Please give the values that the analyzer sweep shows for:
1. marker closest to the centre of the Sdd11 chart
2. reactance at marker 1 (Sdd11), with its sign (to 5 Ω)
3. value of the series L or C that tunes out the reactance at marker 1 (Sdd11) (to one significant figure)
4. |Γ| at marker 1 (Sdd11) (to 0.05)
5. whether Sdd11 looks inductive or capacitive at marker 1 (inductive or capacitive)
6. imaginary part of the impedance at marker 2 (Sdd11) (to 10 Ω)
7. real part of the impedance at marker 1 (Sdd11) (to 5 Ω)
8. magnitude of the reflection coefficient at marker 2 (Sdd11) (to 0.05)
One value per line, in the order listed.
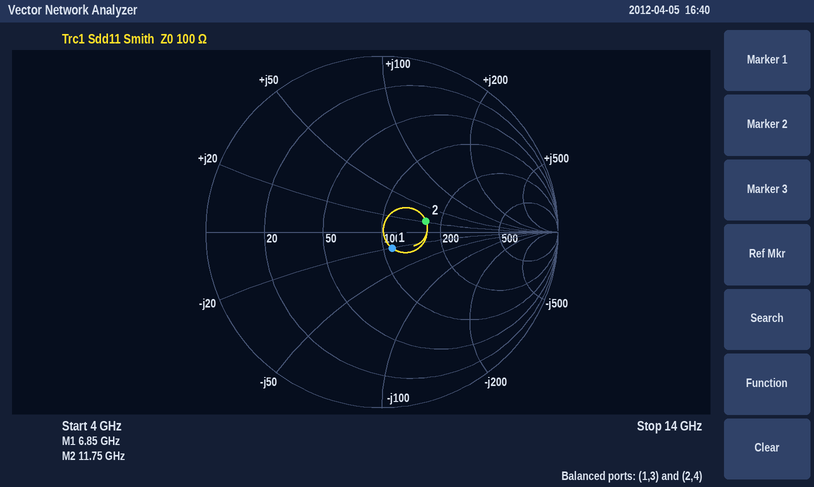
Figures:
marker 1
-20 Ω
500 pH
0.10
capacitive
+20 Ω
110 Ω
0.25
